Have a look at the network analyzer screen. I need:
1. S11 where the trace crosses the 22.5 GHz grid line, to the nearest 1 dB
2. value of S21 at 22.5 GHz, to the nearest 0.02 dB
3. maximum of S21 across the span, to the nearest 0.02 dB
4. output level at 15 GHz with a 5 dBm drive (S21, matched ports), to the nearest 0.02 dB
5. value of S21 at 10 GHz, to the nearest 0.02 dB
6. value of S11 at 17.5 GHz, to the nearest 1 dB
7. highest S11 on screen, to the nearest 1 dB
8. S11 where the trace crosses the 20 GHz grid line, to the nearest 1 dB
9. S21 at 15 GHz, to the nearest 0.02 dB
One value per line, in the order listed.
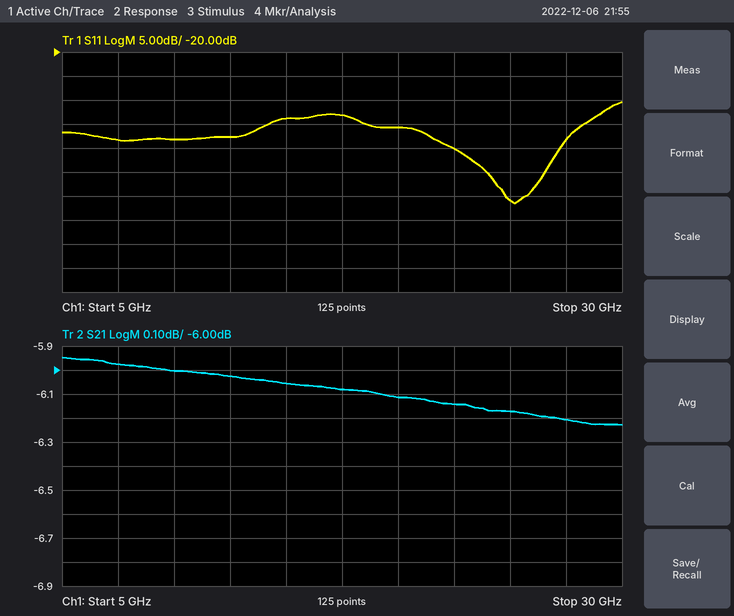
-40 dB
-6.14 dB
-5.94 dB
-1.06 dBm
-6.00 dB
-33 dB
-30 dB
-36 dB
-6.06 dB
